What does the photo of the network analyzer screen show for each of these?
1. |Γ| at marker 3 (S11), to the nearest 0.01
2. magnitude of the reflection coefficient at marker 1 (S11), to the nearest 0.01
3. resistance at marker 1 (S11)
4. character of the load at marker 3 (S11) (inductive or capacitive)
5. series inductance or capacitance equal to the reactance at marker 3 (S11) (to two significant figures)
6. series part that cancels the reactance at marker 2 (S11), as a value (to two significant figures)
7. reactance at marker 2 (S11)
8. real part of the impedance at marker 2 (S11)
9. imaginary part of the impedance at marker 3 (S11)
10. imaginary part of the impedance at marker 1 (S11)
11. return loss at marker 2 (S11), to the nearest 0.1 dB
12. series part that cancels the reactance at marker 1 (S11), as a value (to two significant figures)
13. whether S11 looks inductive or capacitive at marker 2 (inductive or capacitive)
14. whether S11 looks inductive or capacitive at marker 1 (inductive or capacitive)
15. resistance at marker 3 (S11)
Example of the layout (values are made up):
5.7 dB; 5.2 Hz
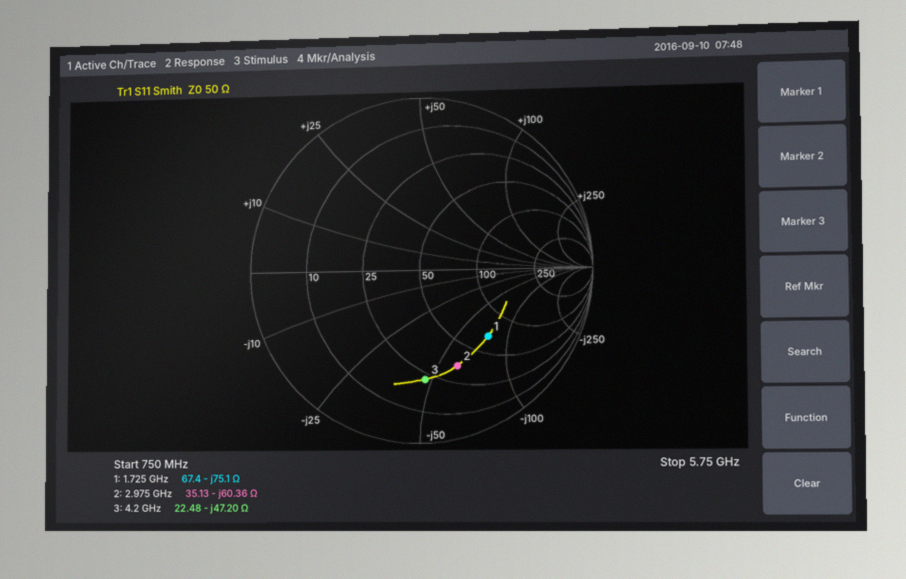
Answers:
0.63; 0.55; 67.4 Ω; capacitive; 800 fF; 3.2 nH; -60.36 Ω; 35.13 Ω; -47.20 Ω; -75.1 Ω; 4.5 dB; 6.9 nH; capacitive; capacitive; 22.48 Ω
